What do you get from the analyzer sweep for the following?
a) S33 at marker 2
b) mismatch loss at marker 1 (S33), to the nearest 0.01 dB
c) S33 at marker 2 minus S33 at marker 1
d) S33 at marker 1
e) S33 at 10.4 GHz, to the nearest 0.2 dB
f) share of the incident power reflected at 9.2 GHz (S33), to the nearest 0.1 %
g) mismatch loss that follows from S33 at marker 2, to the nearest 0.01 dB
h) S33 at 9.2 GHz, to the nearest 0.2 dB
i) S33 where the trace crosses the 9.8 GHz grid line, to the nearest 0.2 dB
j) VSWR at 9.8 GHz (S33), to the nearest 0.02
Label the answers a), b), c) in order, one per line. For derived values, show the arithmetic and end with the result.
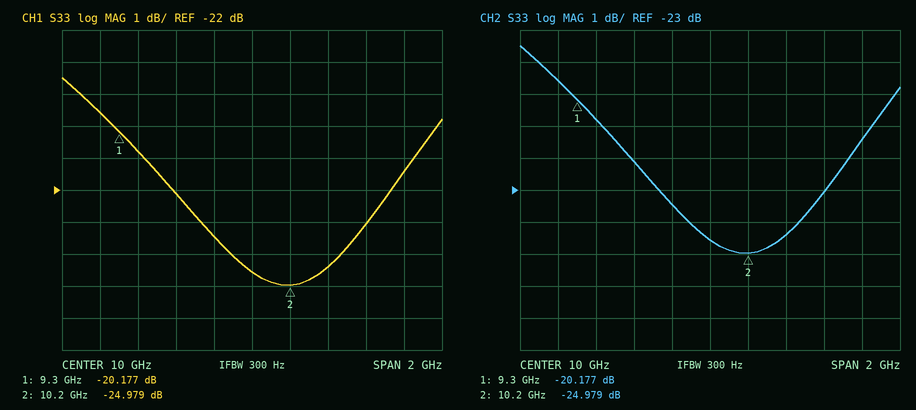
a) -24.979 dB
b) −10 log10(1 − 10^(-20.177/10)) ≈ 0.04 dB
c) -24.979 − (-20.177) = -4.802 dB
d) -20.177 dB
e) -24.4 dB
f) 10^(-19.6/10) ≈ 1.1 %
g) −10 log10(1 − 10^(-24.979/10)) ≈ 0.01 dB
h) -19.6 dB
i) -23.4 dB
j) |Γ| = 10^(-23.4/20) = 0.0676; VSWR = (1 + 0.0676)/(1 − 0.0676) ≈ 1.15, so 1.14 to the nearest 0.02
